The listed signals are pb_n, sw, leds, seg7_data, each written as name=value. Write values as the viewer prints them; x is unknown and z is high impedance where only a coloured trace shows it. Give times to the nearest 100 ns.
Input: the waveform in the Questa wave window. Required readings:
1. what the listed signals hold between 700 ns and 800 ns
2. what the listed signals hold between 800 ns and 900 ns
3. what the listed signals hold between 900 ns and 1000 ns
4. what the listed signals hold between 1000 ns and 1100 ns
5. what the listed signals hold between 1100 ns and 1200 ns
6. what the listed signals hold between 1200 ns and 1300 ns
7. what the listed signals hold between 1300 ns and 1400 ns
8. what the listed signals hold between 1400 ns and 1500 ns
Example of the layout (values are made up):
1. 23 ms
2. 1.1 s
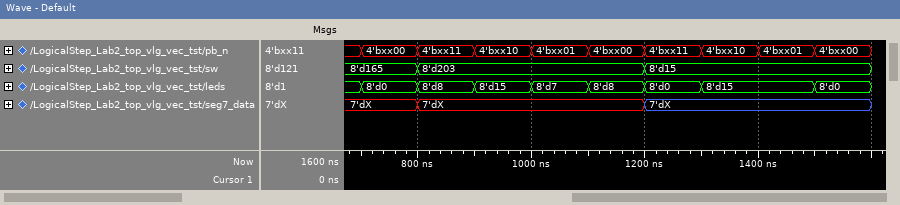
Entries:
1. pb_n=4'bxx00, sw=8'd165, leds=8'd0, seg7_data=7'dX
2. pb_n=4'bxx11, sw=8'd203, leds=8'd8, seg7_data=7'dX
3. pb_n=4'bxx10, sw=8'd203, leds=8'd15, seg7_data=7'dX
4. pb_n=4'bxx01, sw=8'd203, leds=8'd7, seg7_data=7'dX
5. pb_n=4'bxx00, sw=8'd203, leds=8'd8, seg7_data=7'dX
6. pb_n=4'bxx11, sw=8'd15, leds=8'd0, seg7_data=7'dX
7. pb_n=4'bxx10, sw=8'd15, leds=8'd15, seg7_data=7'dX
8. pb_n=4'bxx01, sw=8'd15, leds=8'd15, seg7_data=7'dX
